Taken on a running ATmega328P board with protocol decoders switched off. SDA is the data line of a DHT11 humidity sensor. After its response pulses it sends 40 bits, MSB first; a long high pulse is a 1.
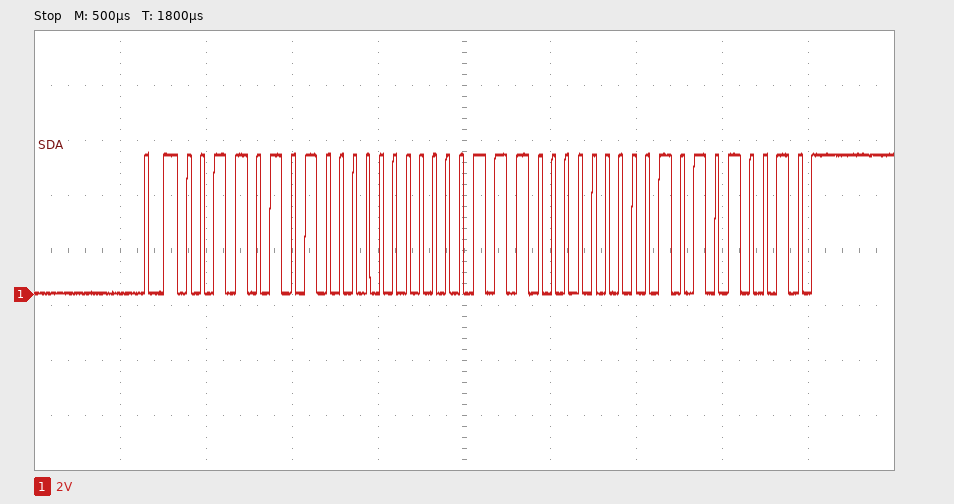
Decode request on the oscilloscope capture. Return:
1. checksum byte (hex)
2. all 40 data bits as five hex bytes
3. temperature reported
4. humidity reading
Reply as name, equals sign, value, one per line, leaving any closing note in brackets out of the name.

checksum byte = 0x52
all 40 data bits as five hex bytes = 35 00 1C 01 52
temperature reported = 28.1 °C
humidity reading = 53 %
